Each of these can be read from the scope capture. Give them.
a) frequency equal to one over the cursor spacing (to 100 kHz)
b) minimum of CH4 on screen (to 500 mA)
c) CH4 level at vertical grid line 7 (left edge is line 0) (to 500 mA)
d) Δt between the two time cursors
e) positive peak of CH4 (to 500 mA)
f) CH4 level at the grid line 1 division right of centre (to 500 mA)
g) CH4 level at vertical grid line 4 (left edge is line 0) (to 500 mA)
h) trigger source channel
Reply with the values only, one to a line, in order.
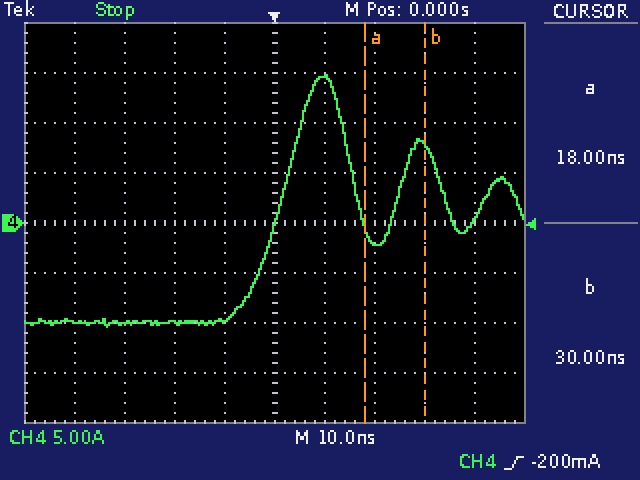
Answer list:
83.3 MHz
-10.5 A
-2.0 A
12 ns
15.0 A
14.5 A
-10.0 A
CH4
